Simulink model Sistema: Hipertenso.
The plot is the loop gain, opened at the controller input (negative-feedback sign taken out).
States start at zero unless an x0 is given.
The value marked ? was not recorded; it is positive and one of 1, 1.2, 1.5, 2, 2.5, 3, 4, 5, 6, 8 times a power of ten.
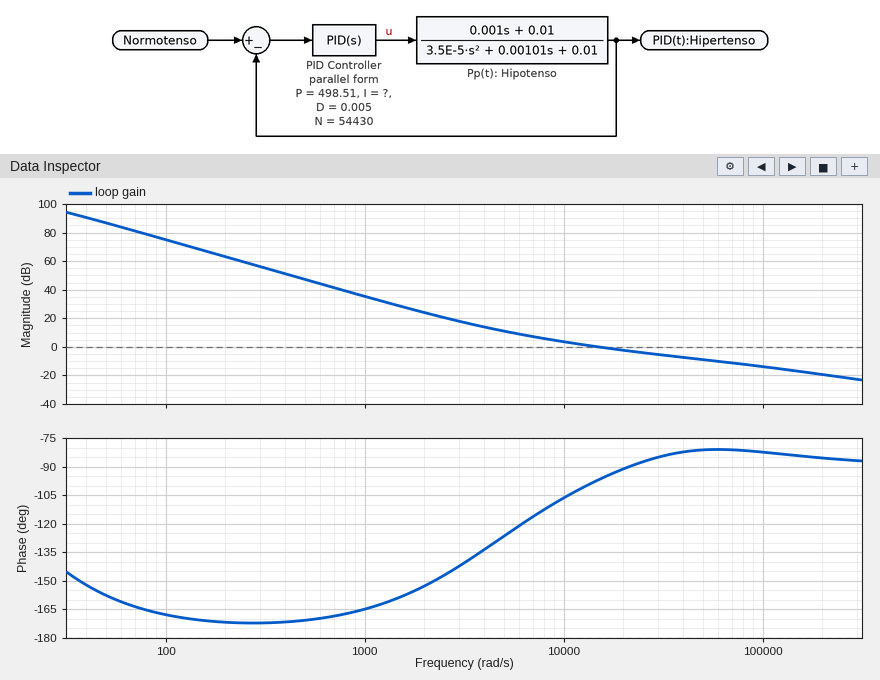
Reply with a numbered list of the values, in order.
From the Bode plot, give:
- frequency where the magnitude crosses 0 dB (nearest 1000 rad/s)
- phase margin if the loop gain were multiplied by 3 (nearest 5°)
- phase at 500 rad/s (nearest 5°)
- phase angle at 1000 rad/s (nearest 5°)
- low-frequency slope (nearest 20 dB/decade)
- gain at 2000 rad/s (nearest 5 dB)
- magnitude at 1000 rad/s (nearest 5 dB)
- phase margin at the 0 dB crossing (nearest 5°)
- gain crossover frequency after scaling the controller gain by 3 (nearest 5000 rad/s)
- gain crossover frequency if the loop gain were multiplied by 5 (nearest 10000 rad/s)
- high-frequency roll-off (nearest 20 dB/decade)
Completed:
1. 15000 rad/s
2. 100°
3. -170°
4. -165°
5. -40 dB/decade
6. 25 dB
7. 35 dB
8. 85°
9. 55000 rad/s
10. 100000 rad/s
11. -20 dB/decade
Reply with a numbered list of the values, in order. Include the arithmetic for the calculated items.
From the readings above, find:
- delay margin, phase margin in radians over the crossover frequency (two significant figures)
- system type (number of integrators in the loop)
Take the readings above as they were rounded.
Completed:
1. 85 × π / 180 / 15000 = 0.000099 s
2. 2
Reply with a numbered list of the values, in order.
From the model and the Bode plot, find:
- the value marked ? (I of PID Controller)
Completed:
1. 2e+06
